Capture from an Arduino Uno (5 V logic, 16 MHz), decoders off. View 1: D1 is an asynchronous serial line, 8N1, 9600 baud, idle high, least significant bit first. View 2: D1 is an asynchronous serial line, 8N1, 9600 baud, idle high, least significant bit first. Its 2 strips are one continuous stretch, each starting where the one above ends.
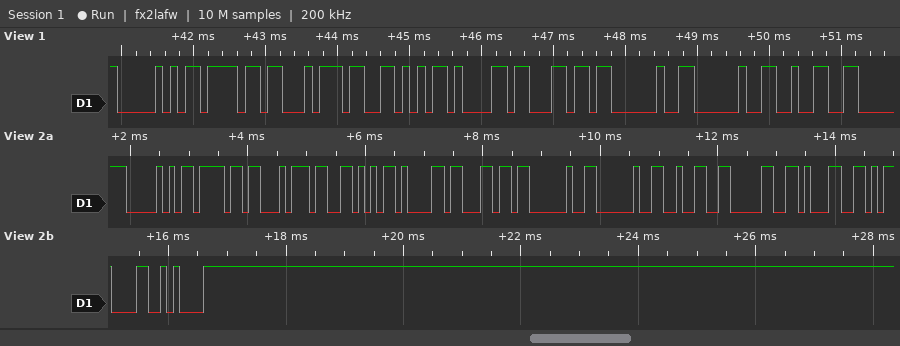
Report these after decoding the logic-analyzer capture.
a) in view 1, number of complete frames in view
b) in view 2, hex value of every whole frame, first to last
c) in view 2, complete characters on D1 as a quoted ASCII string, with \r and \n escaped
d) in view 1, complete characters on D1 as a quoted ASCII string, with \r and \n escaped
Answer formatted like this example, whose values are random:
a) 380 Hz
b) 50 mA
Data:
a) 9
b) 50 6F 74 56 61 6C 20 20 32 30 31 0D 0A
c) "PotVal  201\r\n"
d) "PotVal  2"
